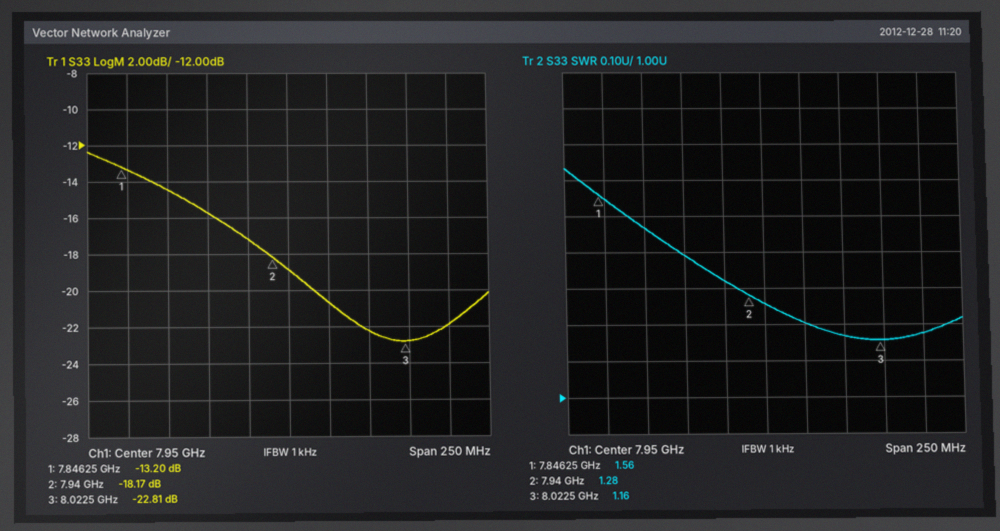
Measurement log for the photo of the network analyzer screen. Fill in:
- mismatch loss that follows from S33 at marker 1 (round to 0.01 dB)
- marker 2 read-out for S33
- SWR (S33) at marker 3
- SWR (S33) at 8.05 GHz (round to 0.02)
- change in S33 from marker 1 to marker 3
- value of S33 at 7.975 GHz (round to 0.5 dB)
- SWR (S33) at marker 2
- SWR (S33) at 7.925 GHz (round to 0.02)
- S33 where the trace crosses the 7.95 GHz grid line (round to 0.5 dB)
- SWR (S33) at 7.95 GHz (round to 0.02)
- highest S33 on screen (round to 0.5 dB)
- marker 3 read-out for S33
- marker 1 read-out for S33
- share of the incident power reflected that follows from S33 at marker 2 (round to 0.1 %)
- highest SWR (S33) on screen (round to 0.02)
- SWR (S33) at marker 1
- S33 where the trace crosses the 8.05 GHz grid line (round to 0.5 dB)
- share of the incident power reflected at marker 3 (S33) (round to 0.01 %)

0.21 dB
-18.17 dB
1.16
1.18
-9.61 dB
-20.5 dB
1.28
1.32
-19.0 dB
1.26
-12.5 dB
-22.81 dB
-13.20 dB
1.5 %
1.64
1.56
-22.0 dB
0.52 %
